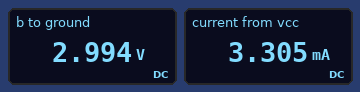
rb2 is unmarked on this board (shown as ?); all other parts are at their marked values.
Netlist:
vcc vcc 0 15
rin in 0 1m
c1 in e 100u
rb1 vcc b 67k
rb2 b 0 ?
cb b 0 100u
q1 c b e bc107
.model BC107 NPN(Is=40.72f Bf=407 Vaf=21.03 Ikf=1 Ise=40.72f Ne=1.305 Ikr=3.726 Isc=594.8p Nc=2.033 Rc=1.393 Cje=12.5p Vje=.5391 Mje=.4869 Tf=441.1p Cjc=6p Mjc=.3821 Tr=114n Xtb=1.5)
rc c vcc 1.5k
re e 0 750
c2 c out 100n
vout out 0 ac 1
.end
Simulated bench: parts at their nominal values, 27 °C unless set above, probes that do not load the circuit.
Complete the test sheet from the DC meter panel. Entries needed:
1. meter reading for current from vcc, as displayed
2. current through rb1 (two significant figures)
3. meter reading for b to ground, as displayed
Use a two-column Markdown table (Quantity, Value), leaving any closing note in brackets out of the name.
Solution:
| Quantity | Value |
|---|---|
| meter reading for current from vcc, as displayed | 3.305 mA |
| current through rb1 | 180 µA |
| meter reading for b to ground, as displayed | 2.994 V |
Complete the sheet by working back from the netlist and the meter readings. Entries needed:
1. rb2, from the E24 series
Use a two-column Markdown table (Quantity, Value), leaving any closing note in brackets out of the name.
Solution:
| Quantity | Value |
|---|---|
| rb2, from the E24 series | 18 kΩ |
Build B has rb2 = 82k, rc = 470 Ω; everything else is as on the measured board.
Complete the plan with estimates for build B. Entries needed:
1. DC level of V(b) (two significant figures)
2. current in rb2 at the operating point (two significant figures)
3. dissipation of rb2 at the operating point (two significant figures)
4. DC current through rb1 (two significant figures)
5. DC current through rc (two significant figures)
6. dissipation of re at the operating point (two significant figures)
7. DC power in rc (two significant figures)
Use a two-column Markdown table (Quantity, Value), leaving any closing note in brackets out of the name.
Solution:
| Quantity | Value |
|---|---|
| DC level of V(b) | 7.0 V |
| current in rb2 at the operating point | 85 µA |
| dissipation of rb2 at the operating point | 600 µW |
| DC current through rb1 | 120 µA |
| DC current through rc | 8.4 mA |
| dissipation of re at the operating point | 53 mW |
| DC power in rc | 33 mW |
